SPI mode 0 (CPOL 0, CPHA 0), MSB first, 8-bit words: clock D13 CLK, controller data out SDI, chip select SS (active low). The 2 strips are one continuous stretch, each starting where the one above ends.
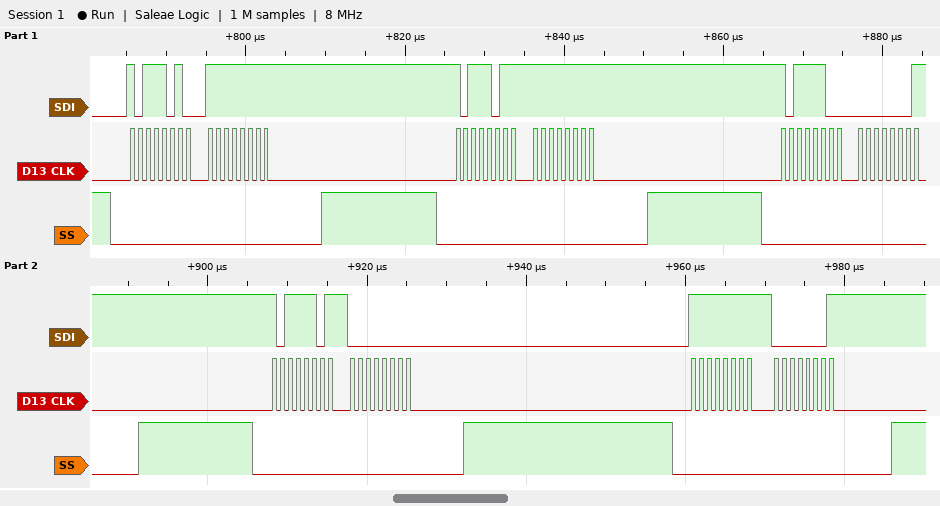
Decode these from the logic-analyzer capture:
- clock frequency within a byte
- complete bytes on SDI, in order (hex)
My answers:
1 MHz
0xBA 0xFF 0xBB 0xFF 0xBC 0x01 0xBD 0x00 0xFF 0x01
